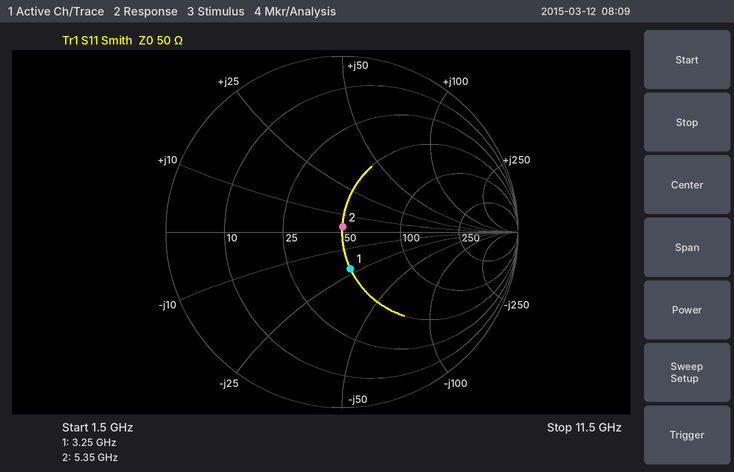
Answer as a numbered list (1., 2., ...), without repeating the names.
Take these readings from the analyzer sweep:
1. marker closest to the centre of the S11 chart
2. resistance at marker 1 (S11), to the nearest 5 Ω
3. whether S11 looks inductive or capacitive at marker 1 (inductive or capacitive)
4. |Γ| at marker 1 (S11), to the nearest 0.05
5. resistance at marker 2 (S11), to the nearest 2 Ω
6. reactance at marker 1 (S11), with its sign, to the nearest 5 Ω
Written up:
1. marker 2
2. 50 Ω
3. capacitive
4. 0.20
5. 50 Ω
6. -20 Ω
